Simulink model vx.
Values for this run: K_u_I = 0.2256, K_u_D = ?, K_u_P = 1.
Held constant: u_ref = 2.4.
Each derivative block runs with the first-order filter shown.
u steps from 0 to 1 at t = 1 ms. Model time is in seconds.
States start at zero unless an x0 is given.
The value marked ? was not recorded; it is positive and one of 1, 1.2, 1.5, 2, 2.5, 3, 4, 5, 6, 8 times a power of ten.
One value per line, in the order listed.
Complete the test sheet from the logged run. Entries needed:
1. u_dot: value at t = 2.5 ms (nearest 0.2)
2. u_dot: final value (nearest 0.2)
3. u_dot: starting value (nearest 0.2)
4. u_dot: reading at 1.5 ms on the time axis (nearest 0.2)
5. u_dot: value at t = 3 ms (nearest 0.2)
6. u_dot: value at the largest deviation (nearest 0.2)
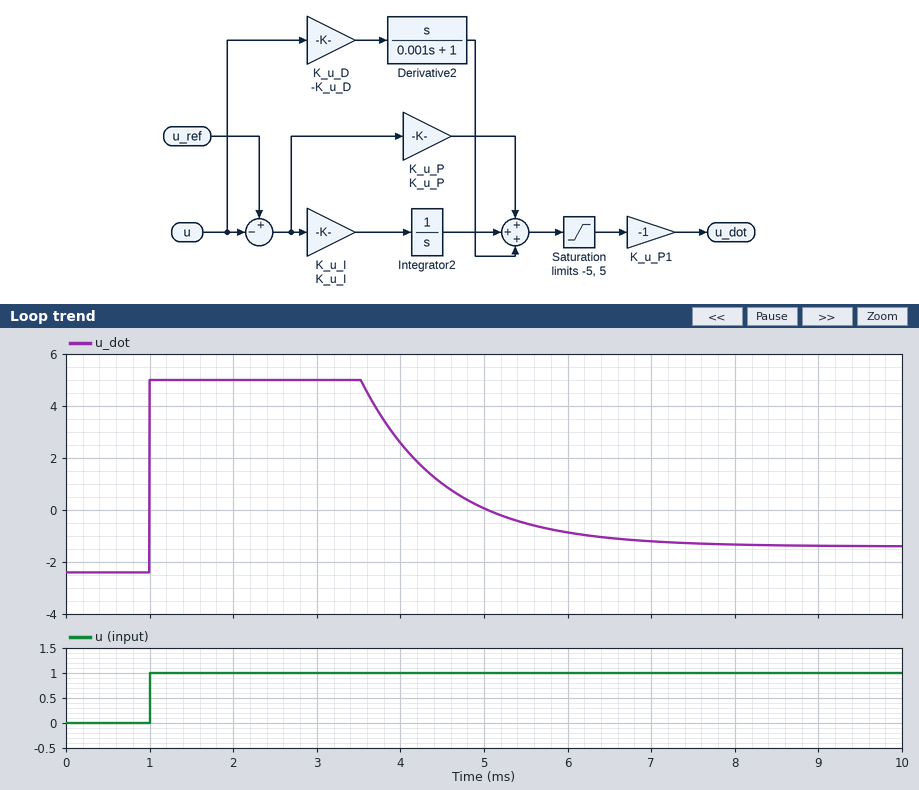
5.0
-1.4
-2.4
5.0
5.0
5.0
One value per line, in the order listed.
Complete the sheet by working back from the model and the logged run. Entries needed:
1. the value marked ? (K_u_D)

0.08
